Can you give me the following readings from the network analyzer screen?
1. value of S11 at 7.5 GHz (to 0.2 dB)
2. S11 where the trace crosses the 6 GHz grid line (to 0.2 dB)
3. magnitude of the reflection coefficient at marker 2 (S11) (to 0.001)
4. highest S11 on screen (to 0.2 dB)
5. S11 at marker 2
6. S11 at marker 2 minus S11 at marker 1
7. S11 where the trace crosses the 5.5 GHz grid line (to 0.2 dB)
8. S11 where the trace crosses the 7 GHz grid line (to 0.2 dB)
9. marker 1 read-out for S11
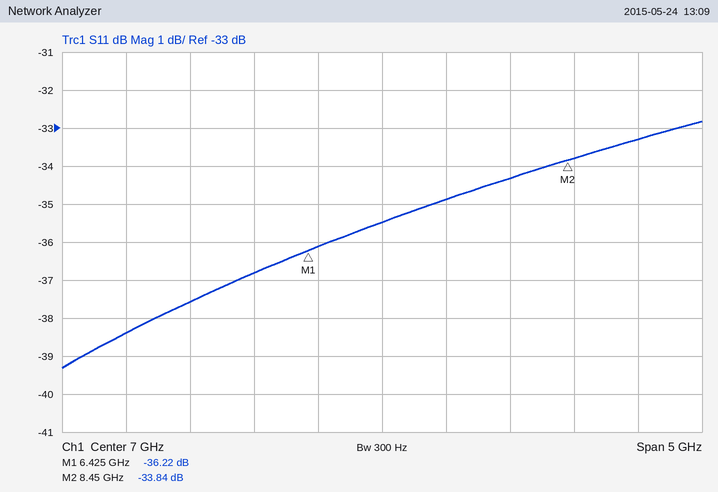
-34.8 dB
-36.8 dB
0.020
-32.8 dB
-33.84 dB
2.38 dB
-37.6 dB
-35.4 dB
-36.22 dB
